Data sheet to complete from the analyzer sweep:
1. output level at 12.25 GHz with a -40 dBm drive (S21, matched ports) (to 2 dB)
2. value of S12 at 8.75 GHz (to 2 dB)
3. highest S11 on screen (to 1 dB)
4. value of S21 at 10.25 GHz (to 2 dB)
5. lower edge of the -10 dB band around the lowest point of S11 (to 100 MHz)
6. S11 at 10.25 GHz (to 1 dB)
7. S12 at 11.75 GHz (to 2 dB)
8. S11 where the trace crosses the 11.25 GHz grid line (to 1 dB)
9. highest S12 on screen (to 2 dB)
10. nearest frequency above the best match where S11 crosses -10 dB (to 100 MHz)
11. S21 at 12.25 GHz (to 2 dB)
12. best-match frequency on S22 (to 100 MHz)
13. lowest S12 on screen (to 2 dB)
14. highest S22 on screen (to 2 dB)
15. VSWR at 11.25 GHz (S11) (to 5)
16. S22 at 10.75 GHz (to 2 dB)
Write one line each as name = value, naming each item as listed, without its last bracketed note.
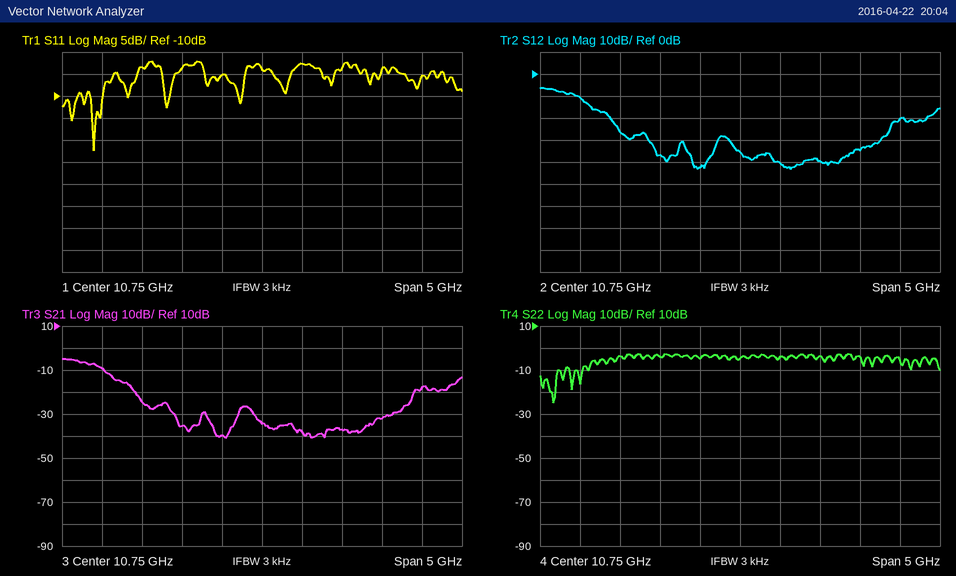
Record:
output level at 12.25 GHz with a -40 dBm drive (S21, matched ports) = -72 dBm
value of S12 at 8.75 GHz = -10 dB
highest S11 on screen = -2 dB
value of S21 at 10.25 GHz = -40 dB
lower edge of the -10 dB band around the lowest point of S11 = 8.6 GHz
S11 at 10.25 GHz = -5 dB
S12 at 11.75 GHz = -40 dB
S11 where the trace crosses the 11.25 GHz grid line = -3 dB
highest S12 on screen = -6 dB
nearest frequency above the best match where S11 crosses -10 dB = 8.8 GHz
S21 at 12.25 GHz = -32 dB
best-match frequency on S22 = 8.4 GHz
lowest S12 on screen = -44 dB
highest S22 on screen = -2 dB
VSWR at 11.25 GHz (S11) = 5
S22 at 10.75 GHz = -4 dB
